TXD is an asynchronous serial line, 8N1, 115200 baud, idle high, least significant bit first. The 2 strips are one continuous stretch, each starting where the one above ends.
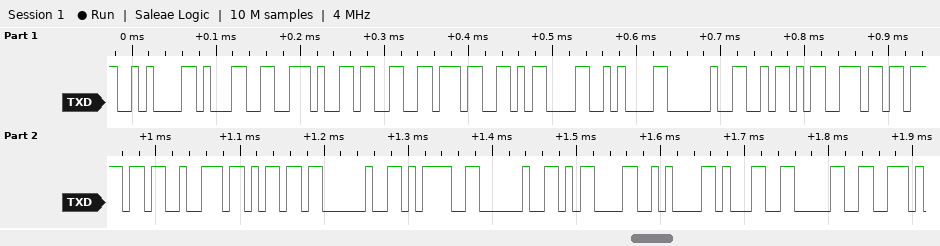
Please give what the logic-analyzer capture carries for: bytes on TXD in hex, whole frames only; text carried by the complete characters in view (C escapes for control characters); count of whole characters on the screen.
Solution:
0A 31 2E 33 37 0D 0A 20 5A 6E 6F 72 6D 20 3D 20 0D 0A 31 30
"\n1.37\r\n Znorm = \r\n10"
20
